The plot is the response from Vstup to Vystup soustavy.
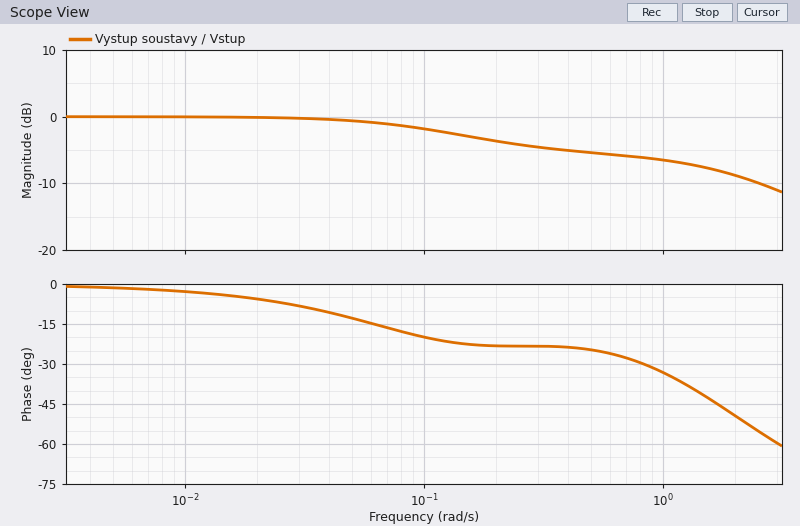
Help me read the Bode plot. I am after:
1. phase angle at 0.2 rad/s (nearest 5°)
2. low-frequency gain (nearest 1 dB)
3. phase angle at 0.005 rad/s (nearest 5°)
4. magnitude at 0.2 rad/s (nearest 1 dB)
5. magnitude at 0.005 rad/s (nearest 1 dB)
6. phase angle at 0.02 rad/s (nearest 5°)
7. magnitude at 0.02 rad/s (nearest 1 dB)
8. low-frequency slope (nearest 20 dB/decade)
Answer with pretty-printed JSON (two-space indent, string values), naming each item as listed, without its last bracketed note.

{
  "phase angle at 0.2 rad/s": "-25°",
  "low-frequency gain": "0 dB",
  "phase angle at 0.005 rad/s": "0°",
  "magnitude at 0.2 rad/s": "-4 dB",
  "magnitude at 0.005 rad/s": "0 dB",
  "phase angle at 0.02 rad/s": "-5°",
  "magnitude at 0.02 rad/s": "0 dB",
  "low-frequency slope": "0 dB/decade"
}
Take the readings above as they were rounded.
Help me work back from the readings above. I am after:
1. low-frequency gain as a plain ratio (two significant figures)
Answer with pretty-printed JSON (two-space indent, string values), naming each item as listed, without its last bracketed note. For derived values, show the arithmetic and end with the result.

{
  "low-frequency gain as a plain ratio": "10^(0 / 20) = 1.0"
}
